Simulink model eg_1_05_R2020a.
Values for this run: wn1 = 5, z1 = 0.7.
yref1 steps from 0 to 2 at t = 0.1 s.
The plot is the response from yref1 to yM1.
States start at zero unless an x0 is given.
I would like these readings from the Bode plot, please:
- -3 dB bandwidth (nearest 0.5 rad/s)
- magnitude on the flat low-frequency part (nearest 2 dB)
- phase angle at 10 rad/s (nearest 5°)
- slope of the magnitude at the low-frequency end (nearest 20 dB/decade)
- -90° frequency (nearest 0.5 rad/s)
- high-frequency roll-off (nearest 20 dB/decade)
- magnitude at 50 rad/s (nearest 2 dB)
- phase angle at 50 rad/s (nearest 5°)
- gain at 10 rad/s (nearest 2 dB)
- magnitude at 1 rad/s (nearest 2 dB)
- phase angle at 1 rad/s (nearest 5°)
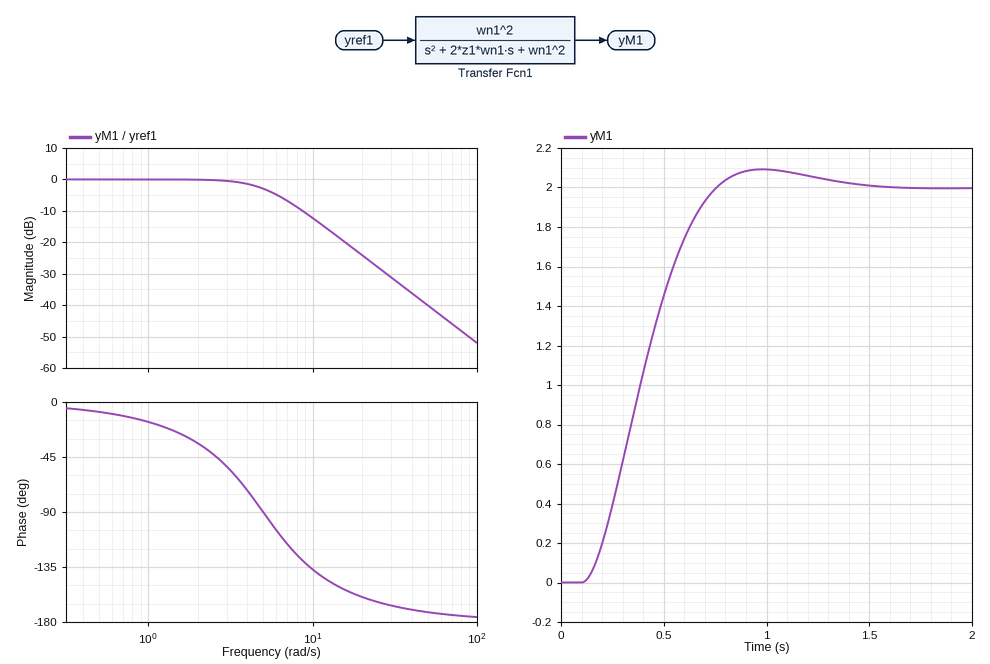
5.0 rad/s
0 dB
-135°
0 dB/decade
5.0 rad/s
-40 dB/decade
-40 dB
-170°
-12 dB
0 dB
-15°
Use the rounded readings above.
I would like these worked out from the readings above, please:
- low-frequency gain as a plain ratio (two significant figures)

1.0
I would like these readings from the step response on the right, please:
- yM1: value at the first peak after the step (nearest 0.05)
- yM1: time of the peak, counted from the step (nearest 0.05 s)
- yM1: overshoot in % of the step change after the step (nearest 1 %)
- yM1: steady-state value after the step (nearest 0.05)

2.10
0.90 s
5 %
2.00
